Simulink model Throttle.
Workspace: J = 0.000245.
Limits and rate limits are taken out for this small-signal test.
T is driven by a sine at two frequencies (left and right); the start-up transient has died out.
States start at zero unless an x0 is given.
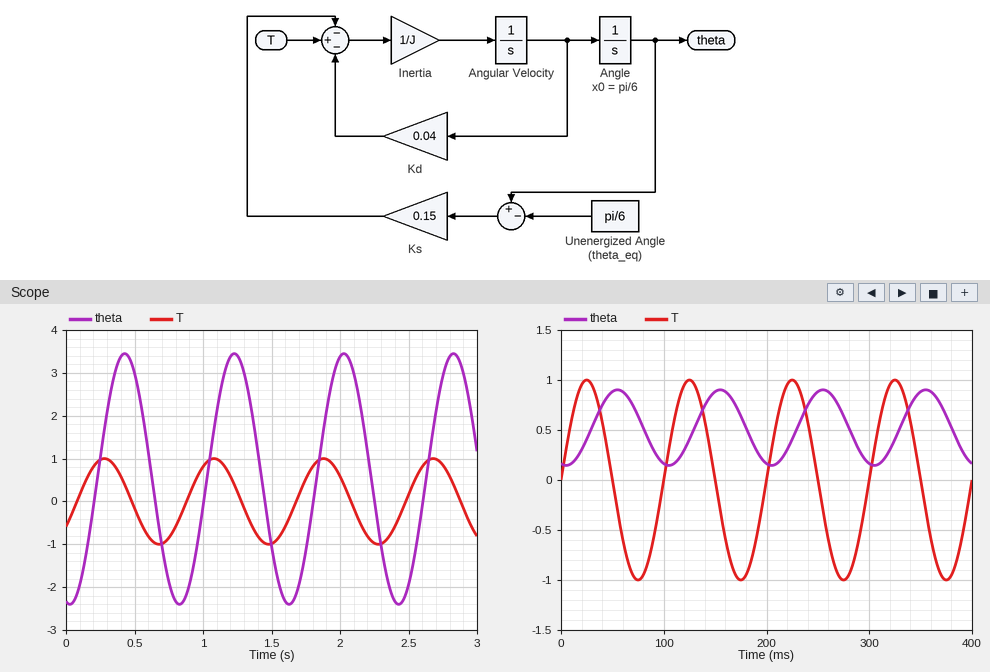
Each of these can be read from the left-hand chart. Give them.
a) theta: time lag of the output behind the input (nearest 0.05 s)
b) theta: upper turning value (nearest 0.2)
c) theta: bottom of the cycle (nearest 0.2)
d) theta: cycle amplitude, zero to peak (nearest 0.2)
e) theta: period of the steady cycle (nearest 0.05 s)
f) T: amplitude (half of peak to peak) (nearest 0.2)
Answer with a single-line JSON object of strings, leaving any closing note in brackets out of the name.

{"theta: time lag of the output behind the input": "0.15 s", "theta: upper turning value": "3.4", "theta: bottom of the cycle": "-2.4", "theta: cycle amplitude, zero to peak": "3.0", "theta: period of the steady cycle": "0.80 s", "T: amplitude (half of peak to peak)": "1.0"}
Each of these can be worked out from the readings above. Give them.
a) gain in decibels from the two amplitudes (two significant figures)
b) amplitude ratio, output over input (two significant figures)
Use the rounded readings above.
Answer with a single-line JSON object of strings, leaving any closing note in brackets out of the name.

{"gain in decibels from the two amplitudes": "9.5 dB", "amplitude ratio, output over input": "3.0"}
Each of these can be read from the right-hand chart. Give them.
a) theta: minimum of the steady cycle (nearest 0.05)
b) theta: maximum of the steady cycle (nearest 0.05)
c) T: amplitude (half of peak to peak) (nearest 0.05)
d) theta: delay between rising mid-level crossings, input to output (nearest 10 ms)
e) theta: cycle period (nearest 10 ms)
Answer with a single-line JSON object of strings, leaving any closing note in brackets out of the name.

{"theta: minimum of the steady cycle": "0.15", "theta: maximum of the steady cycle": "0.90", "T: amplitude (half of peak to peak)": "1.00", "theta: delay between rising mid-level crossings, input to output": "30 ms", "theta: cycle period": "100 ms"}
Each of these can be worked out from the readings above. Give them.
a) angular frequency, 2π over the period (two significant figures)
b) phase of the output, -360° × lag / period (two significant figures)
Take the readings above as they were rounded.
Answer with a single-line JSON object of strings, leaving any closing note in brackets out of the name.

{"angular frequency, 2π over the period": "0.063 rad/ms", "phase of the output, -360° × lag / period": "-110°"}
